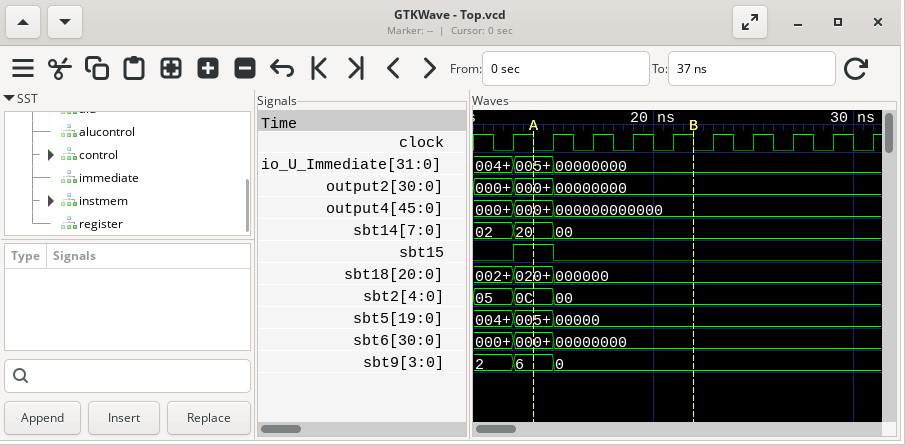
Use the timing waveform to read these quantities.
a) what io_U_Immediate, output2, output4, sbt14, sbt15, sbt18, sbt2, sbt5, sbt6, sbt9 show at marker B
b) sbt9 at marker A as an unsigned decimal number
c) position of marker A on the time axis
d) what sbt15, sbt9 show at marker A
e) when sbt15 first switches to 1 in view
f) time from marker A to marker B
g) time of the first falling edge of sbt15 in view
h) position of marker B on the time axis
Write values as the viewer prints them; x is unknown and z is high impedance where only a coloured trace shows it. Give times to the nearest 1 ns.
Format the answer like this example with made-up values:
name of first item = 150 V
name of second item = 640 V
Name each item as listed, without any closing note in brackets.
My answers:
what io_U_Immediate, output2, output4, sbt14, sbt15, sbt18, sbt2, sbt5, sbt6, sbt9 show at marker B = io_U_Immediate=00000000, output2=00000000, output4=000000000000, sbt14=00, sbt15=0, sbt18=000000, sbt2=00, sbt5=00000, sbt6=00000000, sbt9=0
sbt9 at marker A as an unsigned decimal number = 6
position of marker A on the time axis = 14 ns
what sbt15, sbt9 show at marker A = sbt15=1, sbt9=6
when sbt15 first switches to 1 in view = 13 ns
time from marker A to marker B = 8 ns
time of the first falling edge of sbt15 in view = 15 ns
position of marker B on the time axis = 22 ns
